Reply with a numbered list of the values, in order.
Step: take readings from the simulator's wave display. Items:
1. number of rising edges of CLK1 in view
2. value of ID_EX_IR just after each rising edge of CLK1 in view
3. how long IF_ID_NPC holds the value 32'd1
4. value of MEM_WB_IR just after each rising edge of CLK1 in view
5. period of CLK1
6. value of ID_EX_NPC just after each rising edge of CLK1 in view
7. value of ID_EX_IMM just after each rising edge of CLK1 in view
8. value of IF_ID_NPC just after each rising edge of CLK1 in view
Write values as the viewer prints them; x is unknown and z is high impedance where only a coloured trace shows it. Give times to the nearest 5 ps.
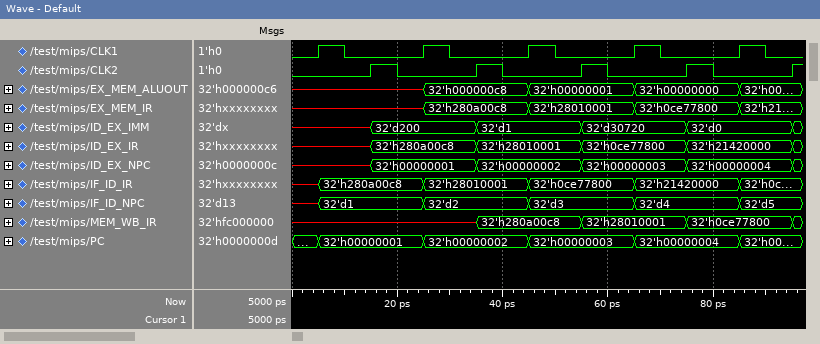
1. 5
2. x, 32'h280a00c8, 32'h28010001, 32'h0ce77800, 32'h21420000
3. 20 ps
4. x, x, 32'h280a00c8, 32'h28010001, 32'h0ce77800
5. 20 ps
6. x, 32'h00000001, 32'h00000002, 32'h00000003, 32'h00000004
7. x, 32'd200, 32'd1, 32'd30720, 32'd0
8. 32'd1, 32'd2, 32'd3, 32'd4, 32'd5
